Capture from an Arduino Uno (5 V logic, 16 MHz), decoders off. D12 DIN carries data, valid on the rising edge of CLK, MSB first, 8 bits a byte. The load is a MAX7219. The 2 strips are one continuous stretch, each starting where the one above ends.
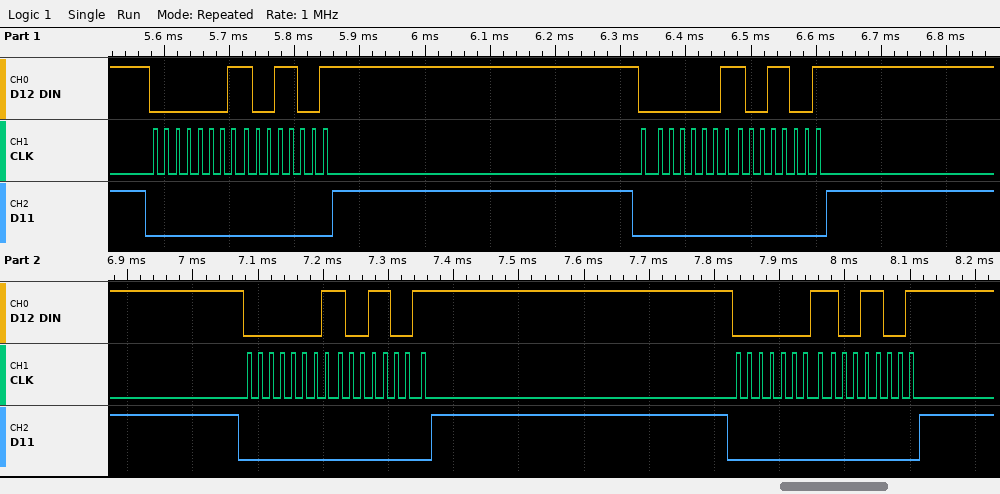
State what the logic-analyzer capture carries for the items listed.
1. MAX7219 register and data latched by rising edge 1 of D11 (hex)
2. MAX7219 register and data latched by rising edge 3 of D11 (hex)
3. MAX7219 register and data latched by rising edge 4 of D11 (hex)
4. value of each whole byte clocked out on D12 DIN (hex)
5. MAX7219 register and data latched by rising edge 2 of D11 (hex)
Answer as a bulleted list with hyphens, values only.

- register 0x1, data 0x99
- register 0x1, data 0x99
- register 0x1, data 0x99
- 01 99 01 99 01 99 01 99
- register 0x1, data 0x99
